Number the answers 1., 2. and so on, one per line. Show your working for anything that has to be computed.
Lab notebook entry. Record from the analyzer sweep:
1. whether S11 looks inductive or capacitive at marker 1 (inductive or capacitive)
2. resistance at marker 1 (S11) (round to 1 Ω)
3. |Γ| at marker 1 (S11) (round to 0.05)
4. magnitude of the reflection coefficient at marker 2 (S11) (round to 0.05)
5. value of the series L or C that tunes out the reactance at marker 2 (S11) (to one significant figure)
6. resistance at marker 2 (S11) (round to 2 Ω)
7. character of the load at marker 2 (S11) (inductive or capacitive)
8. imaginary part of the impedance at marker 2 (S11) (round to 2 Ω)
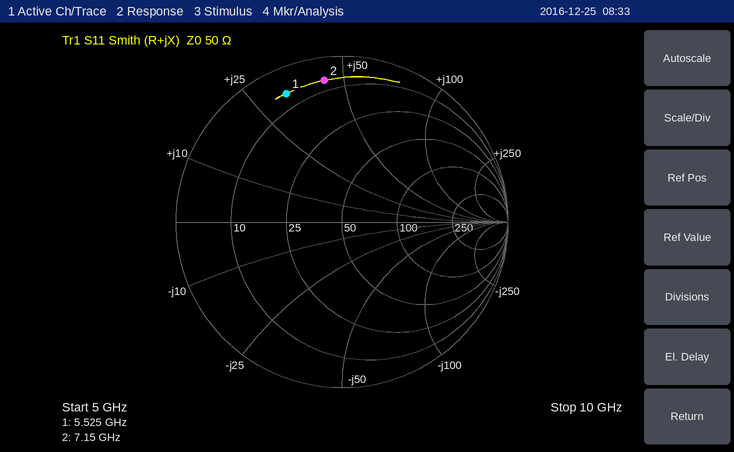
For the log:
1. inductive
2. 6 Ω
3. 0.85
4. 0.85
5. C = 1/(2π × 7.15 GHz × 44 Ω) ≈ 506 fF, so 500 fF to one significant figure
6. 6 Ω
7. inductive
8. +44 Ω
